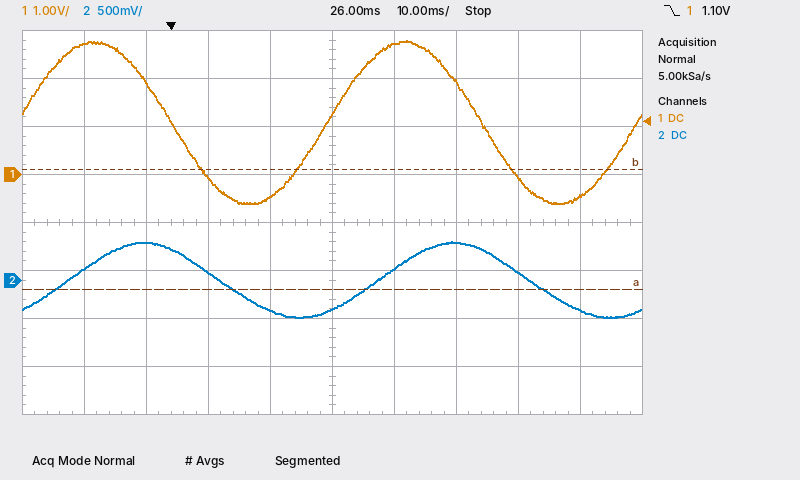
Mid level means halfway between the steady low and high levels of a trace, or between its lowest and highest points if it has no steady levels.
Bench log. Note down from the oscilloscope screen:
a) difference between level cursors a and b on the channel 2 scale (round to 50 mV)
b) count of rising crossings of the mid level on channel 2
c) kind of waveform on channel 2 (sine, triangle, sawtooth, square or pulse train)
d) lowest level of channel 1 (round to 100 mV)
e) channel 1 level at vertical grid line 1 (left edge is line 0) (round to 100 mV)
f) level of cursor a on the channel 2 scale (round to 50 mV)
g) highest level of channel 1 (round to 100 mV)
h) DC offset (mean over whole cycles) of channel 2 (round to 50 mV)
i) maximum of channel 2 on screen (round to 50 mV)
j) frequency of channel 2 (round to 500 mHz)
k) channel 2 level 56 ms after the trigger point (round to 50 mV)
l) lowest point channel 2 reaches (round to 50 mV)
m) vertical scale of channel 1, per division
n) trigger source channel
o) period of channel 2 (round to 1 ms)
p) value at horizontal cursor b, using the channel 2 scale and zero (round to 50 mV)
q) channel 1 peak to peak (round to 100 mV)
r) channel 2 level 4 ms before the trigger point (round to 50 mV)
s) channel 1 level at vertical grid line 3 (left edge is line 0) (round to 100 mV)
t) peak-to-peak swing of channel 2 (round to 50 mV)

1.25 V
2
sine
-600 mV
2.7 V
-100 mV
2.8 V
0 mV
400 mV
20.0 Hz
100 mV
-400 mV
1 V
channel 1
50 ms
1.15 V
3.4 V
400 mV
-100 mV
800 mV
